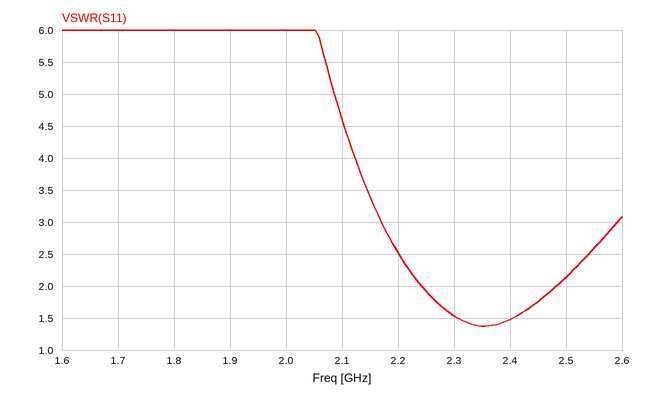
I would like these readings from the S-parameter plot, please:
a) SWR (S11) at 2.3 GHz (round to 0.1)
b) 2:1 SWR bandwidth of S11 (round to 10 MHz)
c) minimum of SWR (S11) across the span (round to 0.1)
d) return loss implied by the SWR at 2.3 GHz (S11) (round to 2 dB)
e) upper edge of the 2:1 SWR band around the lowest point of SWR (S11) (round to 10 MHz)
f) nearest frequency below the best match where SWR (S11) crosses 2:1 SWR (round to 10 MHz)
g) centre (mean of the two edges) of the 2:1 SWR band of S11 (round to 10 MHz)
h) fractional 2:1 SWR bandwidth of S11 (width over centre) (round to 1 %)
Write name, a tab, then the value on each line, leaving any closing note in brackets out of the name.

SWR (S11) at 2.3 GHz	1.5
2:1 SWR bandwidth of S11	240 MHz
minimum of SWR (S11) across the span	1.4
return loss implied by the SWR at 2.3 GHz (S11)	14 dB
upper edge of the 2:1 SWR band around the lowest point of SWR (S11)	2.48 GHz
nearest frequency below the best match where SWR (S11) crosses 2:1 SWR	2.24 GHz
centre (mean of the two edges) of the 2:1 SWR band of S11	2.36 GHz
fractional 2:1 SWR bandwidth of S11 (width over centre)	10 %
